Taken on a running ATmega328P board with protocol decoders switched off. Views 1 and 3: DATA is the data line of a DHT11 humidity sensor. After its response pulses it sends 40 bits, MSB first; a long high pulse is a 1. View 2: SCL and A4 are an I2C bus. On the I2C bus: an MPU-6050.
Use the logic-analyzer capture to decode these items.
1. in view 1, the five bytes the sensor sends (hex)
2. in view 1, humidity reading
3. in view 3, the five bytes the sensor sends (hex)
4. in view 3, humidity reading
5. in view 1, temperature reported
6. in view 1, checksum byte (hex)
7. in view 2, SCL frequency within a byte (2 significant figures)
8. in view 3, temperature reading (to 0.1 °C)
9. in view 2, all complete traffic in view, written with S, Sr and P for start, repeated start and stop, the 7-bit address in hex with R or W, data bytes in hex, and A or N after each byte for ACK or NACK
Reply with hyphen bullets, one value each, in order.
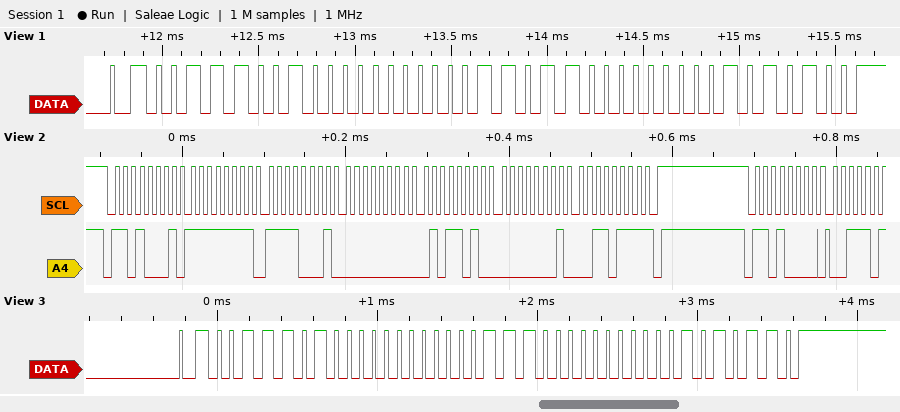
- 39 00 1B 00 54
- 57 %
- 3A 00 1C 00 56
- 58 %
- 27.0 °C
- 0x54
- 100 kHz
- 28.0 °C
- S 68R A FF A F1 A 00 A 5A A 01 A 37 N P S 68W A
